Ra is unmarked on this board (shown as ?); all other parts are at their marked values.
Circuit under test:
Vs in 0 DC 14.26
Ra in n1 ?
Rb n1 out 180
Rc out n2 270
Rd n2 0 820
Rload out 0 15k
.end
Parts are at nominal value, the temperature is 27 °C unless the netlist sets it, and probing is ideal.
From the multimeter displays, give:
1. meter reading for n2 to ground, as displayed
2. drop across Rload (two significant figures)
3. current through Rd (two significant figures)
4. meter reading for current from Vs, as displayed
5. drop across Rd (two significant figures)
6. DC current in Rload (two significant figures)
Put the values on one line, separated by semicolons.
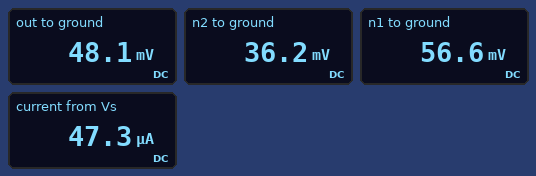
36.2 mV; 48 mV; 44 µA; 47.3 µA; 36 mV; 3.2 µA
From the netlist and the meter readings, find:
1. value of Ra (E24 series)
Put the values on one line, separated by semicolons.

300 kΩ
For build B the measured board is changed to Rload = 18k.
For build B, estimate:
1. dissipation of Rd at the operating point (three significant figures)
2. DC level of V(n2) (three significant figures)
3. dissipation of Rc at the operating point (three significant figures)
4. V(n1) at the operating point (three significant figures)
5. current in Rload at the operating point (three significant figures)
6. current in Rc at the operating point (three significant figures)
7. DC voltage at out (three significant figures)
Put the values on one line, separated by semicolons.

1.63 µW; 36.6 mV; 538 nW; 57.2 mV; 2.70 µA; 44.6 µA; 48.7 mV
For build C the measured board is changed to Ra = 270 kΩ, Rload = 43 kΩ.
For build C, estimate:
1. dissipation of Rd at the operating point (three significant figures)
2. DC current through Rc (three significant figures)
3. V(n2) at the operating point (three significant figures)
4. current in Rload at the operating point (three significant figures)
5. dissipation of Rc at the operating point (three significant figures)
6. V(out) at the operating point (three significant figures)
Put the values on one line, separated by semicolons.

2.16 µW; 51.3 µA; 42.0 mV; 1.30 µA; 710 nW; 55.9 mV
